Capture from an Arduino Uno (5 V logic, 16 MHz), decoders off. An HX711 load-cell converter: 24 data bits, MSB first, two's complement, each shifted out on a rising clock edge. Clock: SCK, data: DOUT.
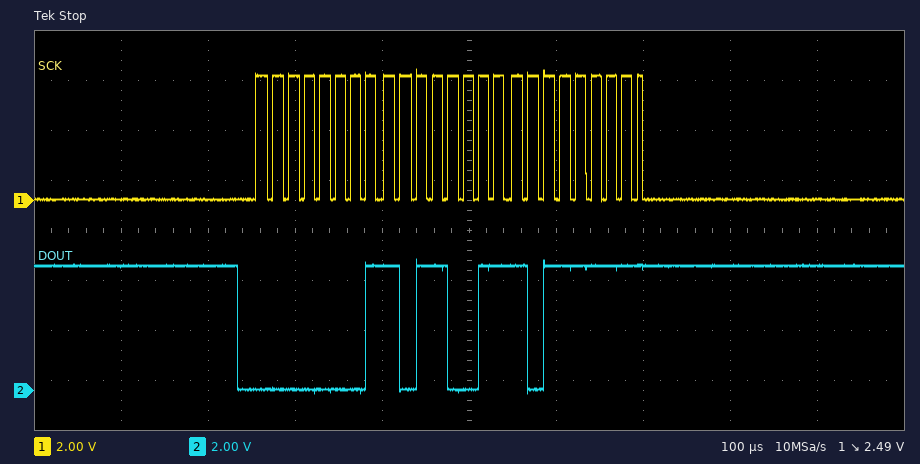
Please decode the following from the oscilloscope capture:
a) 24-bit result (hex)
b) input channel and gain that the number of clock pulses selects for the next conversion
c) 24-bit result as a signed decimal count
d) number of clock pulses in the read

0x01B3BF
channel A, gain 128
111551
25
